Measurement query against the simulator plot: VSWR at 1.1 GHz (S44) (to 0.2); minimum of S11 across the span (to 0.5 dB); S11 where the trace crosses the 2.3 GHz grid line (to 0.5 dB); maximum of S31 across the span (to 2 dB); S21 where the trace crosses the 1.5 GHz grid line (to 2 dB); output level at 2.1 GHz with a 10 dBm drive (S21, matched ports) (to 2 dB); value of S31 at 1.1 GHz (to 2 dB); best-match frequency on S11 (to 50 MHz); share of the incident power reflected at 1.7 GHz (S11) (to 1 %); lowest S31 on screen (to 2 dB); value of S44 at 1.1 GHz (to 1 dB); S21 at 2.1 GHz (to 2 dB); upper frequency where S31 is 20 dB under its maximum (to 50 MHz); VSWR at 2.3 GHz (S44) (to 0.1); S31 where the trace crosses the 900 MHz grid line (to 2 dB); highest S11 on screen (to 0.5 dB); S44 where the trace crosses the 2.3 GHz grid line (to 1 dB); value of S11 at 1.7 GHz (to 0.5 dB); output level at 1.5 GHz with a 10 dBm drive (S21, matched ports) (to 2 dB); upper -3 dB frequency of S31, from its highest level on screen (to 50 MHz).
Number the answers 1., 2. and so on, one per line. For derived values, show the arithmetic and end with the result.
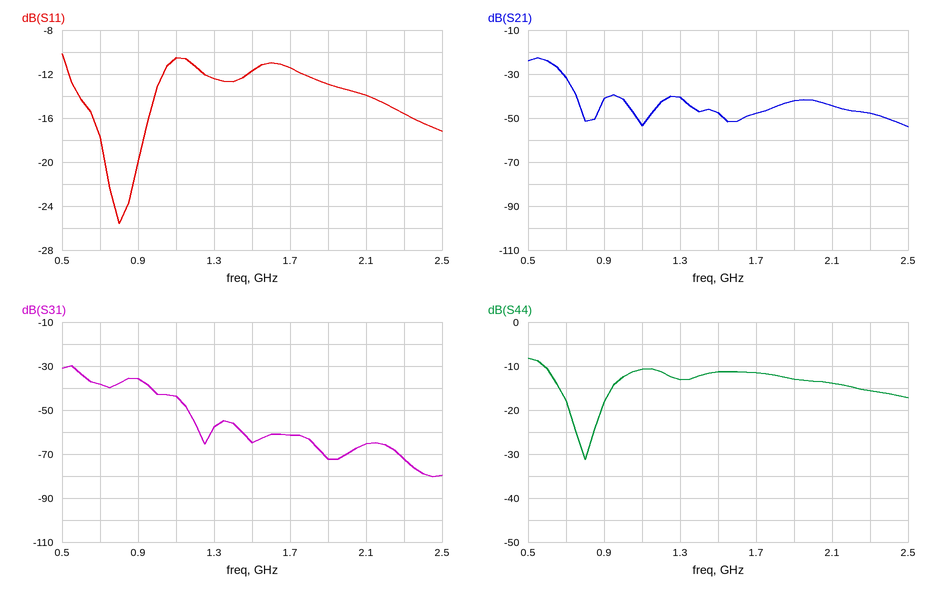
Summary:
1. |Γ| = 10^(-11/20) = 0.2818; VSWR = (1 + 0.2818)/(1 − 0.2818) ≈ 1.8
2. -25.5 dB
3. -15.5 dB
4. -30 dB
5. -48 dB
6. 10 dBm + (-44 dB) = -34 dBm
7. -44 dB
8. 800 MHz
9. 10^(-11.5/10) ≈ 7 %
10. -80 dB
11. -11 dB
12. -44 dB
13. 1.15 GHz
14. |Γ| = 10^(-16/20) = 0.1585; VSWR = (1 + 0.1585)/(1 − 0.1585) ≈ 1.4
15. -36 dB
16. -10.0 dB
17. -16 dB
18. -11.5 dB
19. 10 dBm + (-48 dB) = -38 dBm
20. 600 MHz
